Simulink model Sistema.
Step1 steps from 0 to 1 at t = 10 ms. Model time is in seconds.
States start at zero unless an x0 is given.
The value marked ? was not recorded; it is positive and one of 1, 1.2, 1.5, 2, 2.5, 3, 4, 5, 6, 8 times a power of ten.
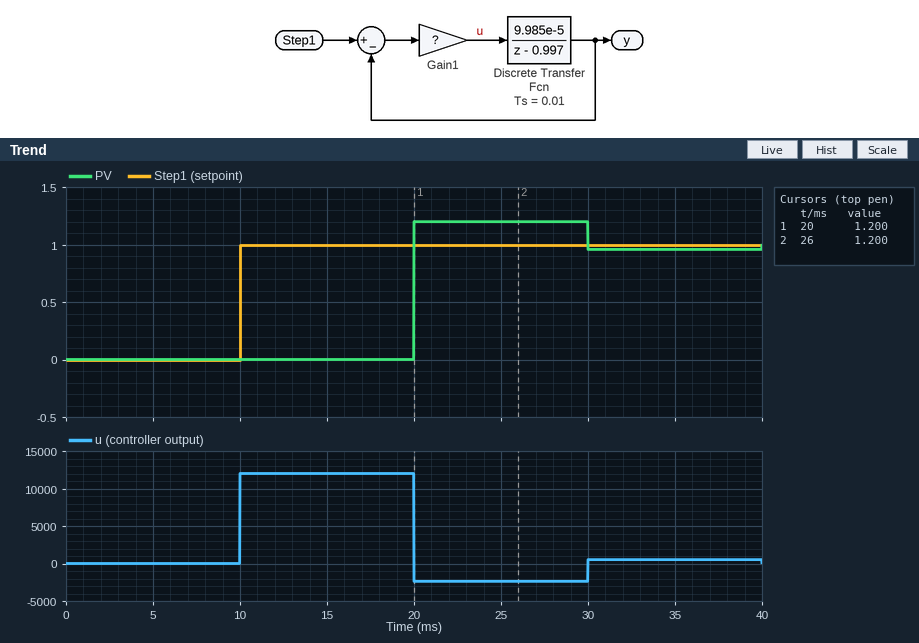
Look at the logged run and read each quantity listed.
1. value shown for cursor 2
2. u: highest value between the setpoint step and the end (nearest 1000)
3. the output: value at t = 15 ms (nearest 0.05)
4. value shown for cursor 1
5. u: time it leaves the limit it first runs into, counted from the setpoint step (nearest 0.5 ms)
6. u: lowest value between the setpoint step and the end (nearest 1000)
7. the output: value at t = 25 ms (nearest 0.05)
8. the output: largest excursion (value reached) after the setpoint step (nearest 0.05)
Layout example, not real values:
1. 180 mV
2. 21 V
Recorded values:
1. 1.200
2. 12000
3. 0.00
4. 1.200
5. 10.0 ms
6. -2000
7. 1.20
8. 1.20
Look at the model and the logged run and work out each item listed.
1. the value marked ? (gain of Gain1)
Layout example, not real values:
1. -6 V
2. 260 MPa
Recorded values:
1. 12000
